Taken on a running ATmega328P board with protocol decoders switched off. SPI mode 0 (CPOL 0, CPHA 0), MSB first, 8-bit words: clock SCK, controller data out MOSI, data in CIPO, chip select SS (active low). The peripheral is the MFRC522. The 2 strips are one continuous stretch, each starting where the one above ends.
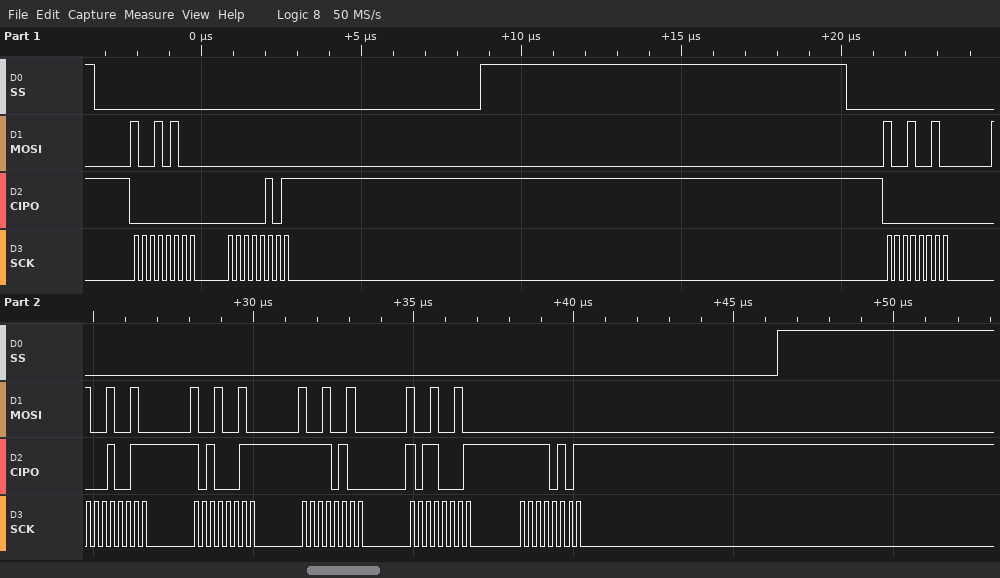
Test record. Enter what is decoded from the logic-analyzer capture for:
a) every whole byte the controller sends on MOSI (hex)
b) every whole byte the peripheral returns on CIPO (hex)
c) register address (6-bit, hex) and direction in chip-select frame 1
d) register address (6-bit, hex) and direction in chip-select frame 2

94 00 92 92 92 92 92 00
00 05 00 13 A3 F4 B1 F5
0x0A read
0x09 read
